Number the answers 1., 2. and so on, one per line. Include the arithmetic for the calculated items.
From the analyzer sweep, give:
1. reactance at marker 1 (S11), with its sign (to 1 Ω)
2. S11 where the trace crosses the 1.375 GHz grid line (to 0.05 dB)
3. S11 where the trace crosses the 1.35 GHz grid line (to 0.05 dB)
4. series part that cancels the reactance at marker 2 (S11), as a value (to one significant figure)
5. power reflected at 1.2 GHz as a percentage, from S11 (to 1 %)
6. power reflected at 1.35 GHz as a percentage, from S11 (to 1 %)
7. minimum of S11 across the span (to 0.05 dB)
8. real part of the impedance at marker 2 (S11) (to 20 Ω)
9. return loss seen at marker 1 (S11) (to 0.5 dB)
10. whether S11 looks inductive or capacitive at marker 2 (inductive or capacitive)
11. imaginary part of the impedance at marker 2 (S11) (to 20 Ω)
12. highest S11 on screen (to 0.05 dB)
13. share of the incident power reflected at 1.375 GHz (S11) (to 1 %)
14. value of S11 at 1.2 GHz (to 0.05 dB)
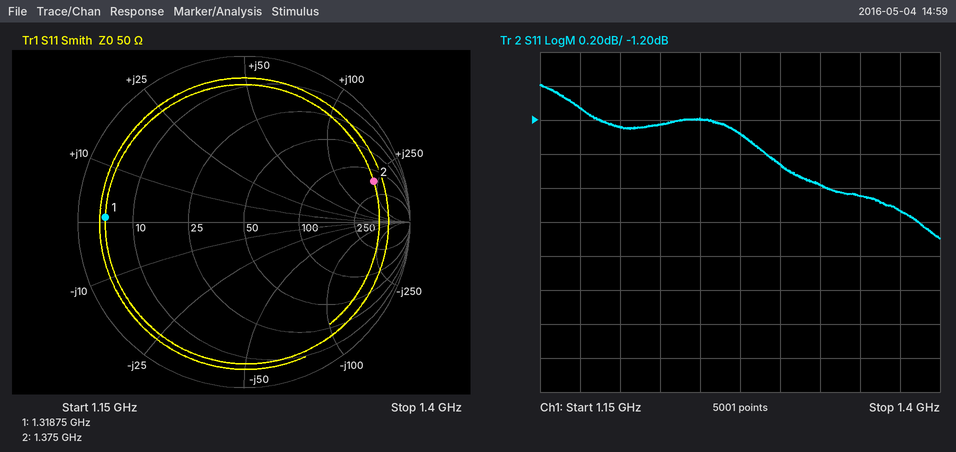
1. +1 Ω
2. -1.75 dB
3. -1.65 dB
4. C = 1/(2π × 1.375 GHz × 220 Ω) ≈ 526 fF, so 500 fF to one significant figure
5. 10^(-1.25/10) ≈ 75 %
6. 10^(-1.65/10) ≈ 68 %
7. -1.90 dB
8. 160 Ω
9. 1.5 dB
10. inductive
11. +220 Ω
12. -1.00 dB
13. 10^(-1.75/10) ≈ 67 %
14. -1.25 dB
